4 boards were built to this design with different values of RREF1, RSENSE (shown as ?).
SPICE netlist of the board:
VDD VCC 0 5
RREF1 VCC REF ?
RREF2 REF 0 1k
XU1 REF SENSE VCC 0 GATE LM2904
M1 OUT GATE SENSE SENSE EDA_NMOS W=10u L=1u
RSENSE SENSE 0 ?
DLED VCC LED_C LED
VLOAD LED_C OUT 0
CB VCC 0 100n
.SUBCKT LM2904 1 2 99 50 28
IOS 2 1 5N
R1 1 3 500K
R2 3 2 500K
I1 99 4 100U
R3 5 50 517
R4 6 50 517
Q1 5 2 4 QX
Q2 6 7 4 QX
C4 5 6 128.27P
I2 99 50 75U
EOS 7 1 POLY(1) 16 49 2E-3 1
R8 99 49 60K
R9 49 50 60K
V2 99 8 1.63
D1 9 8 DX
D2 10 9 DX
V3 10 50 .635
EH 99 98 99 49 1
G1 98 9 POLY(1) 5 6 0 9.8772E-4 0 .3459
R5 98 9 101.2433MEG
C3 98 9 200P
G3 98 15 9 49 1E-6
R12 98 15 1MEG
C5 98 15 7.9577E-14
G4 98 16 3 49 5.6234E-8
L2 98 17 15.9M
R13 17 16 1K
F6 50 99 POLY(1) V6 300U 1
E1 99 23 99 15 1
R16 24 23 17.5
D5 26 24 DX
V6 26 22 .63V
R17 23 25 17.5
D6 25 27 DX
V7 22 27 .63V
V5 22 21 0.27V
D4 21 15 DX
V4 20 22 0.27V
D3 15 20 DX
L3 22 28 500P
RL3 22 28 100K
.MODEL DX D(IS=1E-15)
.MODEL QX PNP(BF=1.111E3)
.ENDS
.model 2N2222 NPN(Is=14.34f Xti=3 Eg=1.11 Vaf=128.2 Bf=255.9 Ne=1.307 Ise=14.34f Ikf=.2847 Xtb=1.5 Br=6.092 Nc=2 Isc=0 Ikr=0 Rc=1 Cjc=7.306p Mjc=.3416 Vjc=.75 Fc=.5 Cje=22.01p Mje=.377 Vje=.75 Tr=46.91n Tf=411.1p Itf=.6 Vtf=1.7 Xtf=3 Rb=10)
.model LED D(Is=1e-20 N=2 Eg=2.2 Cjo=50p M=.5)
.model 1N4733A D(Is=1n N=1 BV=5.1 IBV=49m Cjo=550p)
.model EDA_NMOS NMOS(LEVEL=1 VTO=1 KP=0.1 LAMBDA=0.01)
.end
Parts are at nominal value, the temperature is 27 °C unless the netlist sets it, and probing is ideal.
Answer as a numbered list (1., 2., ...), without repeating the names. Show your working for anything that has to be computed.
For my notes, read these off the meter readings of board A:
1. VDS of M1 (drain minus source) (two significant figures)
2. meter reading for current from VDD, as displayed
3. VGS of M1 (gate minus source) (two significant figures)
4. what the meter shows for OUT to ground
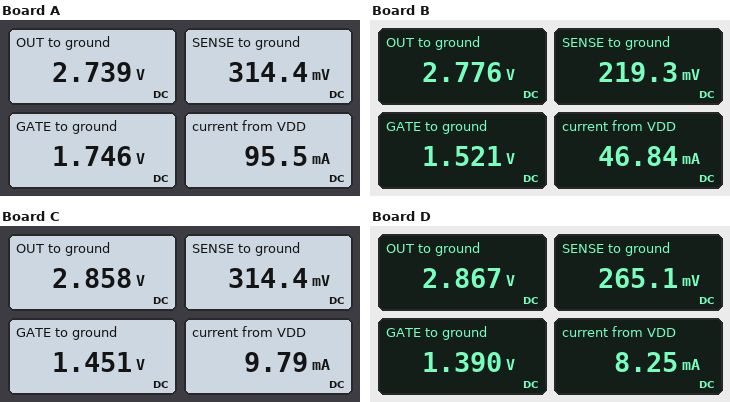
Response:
1. 2.739 V - 314.4 mV = 2.4 V
2. 95.5 mA
3. 1.746 V - 314.4 mV = 1.4 V
4. 2.739 V
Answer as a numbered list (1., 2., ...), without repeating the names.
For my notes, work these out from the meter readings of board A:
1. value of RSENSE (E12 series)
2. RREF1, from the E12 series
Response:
1. 3.3 Ω
2. 15 kΩ
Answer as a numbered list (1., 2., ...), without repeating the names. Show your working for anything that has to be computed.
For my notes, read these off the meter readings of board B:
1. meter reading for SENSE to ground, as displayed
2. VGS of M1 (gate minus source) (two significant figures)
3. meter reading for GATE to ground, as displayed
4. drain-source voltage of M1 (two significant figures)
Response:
1. 219.3 mV
2. 1.521 V - 219.3 mV = 1.3 V
3. 1.521 V
4. 2.776 V - 219.3 mV = 2.6 V
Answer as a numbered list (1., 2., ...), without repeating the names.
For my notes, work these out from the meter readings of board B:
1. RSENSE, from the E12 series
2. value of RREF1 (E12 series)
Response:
1. 4.7 Ω
2. 22 kΩ
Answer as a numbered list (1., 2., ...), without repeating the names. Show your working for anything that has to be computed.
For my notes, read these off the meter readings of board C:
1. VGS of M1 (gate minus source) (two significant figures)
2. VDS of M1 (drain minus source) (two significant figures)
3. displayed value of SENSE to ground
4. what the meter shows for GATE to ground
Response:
1. 1.451 V - 314.4 mV = 1.1 V
2. 2.858 V - 314.4 mV = 2.5 V
3. 314.4 mV
4. 1.451 V
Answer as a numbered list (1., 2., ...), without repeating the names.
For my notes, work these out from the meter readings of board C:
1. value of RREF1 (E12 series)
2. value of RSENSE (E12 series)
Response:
1. 15 kΩ
2. 33 Ω
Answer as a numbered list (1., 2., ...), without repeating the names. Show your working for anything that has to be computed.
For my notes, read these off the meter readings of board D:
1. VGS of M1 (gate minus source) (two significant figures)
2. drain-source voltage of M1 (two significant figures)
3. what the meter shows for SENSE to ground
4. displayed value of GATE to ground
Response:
1. 1.39 V - 265.1 mV = 1.1 V
2. 2.867 V - 265.1 mV = 2.6 V
3. 265.1 mV
4. 1.390 V
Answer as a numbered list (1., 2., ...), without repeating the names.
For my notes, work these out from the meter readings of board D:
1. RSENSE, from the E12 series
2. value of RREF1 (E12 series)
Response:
1. 33 Ω
2. 18 kΩ
